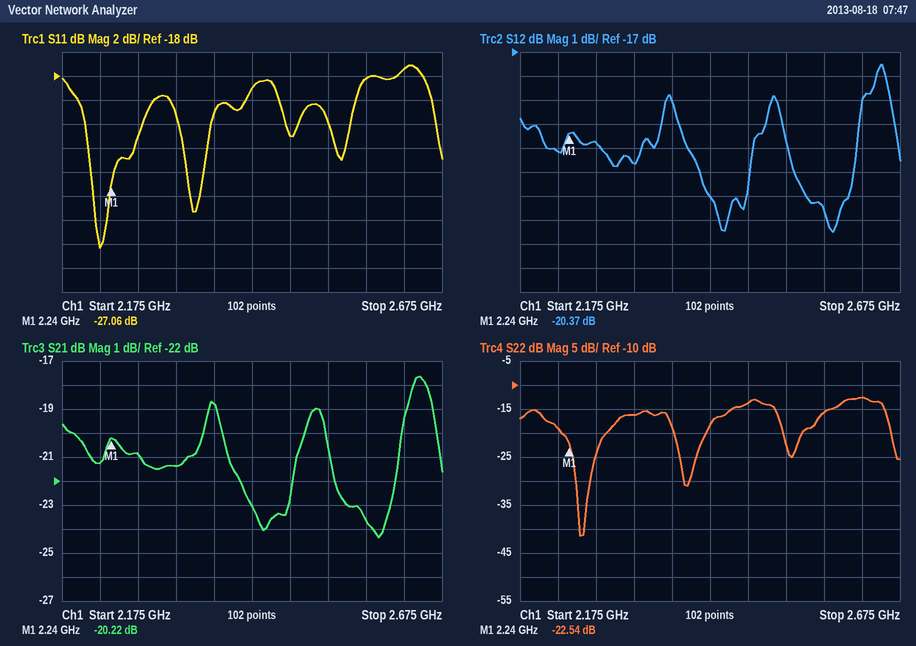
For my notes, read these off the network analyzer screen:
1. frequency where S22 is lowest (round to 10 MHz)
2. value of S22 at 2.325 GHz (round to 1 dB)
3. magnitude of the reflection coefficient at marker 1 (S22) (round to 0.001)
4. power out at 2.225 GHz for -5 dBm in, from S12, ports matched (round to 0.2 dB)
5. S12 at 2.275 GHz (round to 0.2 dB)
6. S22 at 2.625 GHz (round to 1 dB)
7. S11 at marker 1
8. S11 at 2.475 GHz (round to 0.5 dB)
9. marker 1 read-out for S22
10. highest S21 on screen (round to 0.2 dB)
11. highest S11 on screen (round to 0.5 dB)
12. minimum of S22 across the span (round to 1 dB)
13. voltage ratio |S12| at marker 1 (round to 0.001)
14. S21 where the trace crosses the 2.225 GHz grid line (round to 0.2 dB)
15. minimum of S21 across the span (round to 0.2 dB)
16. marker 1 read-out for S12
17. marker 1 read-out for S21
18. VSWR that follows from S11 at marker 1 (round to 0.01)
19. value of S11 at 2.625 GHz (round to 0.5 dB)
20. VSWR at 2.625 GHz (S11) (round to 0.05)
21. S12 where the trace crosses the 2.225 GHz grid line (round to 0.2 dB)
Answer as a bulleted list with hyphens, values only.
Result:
- 2.25 GHz
- -16 dB
- 0.075
- -26.2 dBm
- -20.8 dB
- -13 dB
- -27.06 dB
- -23.0 dB
- -22.54 dB
- -17.6 dB
- -17.0 dB
- -41 dB
- 0.096
- -21.2 dB
- -24.4 dB
- -20.37 dB
- -20.22 dB
- 1.09
- -17.5 dB
- 1.30
- -21.2 dB
